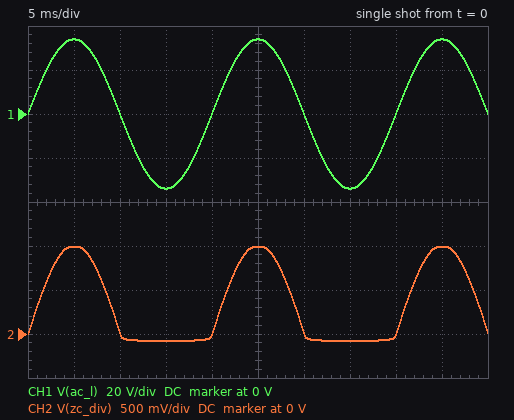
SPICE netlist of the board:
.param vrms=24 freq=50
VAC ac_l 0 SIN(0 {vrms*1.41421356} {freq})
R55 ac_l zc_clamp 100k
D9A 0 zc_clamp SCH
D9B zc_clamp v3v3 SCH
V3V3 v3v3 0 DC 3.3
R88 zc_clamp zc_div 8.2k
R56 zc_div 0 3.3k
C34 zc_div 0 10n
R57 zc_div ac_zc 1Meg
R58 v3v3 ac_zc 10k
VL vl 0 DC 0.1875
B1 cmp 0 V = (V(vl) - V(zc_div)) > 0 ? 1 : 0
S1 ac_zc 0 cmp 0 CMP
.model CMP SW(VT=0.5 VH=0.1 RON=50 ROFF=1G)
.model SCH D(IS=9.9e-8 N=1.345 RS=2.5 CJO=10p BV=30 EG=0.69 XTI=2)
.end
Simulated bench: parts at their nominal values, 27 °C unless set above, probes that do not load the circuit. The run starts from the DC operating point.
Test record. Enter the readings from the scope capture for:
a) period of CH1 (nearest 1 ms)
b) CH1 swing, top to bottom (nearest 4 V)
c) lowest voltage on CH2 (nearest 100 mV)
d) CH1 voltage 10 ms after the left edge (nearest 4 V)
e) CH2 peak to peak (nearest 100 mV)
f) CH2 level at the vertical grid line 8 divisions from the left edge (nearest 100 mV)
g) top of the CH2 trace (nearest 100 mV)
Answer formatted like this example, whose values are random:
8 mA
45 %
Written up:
20 ms
68 V
-100 mV
0 V
1.1 V
0 V
1.0 V
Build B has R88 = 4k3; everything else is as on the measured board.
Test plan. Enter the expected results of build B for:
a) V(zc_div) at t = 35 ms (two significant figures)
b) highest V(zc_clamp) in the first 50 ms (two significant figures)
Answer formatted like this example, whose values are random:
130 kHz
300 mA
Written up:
-120 mV
2.4 V
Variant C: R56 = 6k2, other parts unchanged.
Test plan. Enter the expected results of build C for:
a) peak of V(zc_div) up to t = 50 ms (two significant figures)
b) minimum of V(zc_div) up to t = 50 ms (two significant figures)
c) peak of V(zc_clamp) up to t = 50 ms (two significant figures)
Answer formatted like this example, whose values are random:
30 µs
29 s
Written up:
1.5 V
-120 mV
3.5 V
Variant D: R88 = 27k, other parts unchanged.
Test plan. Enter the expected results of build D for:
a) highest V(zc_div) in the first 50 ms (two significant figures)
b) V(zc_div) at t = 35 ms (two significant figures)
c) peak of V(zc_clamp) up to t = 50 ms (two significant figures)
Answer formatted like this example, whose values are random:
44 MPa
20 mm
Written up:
400 mV
-31 mV
3.6 V
